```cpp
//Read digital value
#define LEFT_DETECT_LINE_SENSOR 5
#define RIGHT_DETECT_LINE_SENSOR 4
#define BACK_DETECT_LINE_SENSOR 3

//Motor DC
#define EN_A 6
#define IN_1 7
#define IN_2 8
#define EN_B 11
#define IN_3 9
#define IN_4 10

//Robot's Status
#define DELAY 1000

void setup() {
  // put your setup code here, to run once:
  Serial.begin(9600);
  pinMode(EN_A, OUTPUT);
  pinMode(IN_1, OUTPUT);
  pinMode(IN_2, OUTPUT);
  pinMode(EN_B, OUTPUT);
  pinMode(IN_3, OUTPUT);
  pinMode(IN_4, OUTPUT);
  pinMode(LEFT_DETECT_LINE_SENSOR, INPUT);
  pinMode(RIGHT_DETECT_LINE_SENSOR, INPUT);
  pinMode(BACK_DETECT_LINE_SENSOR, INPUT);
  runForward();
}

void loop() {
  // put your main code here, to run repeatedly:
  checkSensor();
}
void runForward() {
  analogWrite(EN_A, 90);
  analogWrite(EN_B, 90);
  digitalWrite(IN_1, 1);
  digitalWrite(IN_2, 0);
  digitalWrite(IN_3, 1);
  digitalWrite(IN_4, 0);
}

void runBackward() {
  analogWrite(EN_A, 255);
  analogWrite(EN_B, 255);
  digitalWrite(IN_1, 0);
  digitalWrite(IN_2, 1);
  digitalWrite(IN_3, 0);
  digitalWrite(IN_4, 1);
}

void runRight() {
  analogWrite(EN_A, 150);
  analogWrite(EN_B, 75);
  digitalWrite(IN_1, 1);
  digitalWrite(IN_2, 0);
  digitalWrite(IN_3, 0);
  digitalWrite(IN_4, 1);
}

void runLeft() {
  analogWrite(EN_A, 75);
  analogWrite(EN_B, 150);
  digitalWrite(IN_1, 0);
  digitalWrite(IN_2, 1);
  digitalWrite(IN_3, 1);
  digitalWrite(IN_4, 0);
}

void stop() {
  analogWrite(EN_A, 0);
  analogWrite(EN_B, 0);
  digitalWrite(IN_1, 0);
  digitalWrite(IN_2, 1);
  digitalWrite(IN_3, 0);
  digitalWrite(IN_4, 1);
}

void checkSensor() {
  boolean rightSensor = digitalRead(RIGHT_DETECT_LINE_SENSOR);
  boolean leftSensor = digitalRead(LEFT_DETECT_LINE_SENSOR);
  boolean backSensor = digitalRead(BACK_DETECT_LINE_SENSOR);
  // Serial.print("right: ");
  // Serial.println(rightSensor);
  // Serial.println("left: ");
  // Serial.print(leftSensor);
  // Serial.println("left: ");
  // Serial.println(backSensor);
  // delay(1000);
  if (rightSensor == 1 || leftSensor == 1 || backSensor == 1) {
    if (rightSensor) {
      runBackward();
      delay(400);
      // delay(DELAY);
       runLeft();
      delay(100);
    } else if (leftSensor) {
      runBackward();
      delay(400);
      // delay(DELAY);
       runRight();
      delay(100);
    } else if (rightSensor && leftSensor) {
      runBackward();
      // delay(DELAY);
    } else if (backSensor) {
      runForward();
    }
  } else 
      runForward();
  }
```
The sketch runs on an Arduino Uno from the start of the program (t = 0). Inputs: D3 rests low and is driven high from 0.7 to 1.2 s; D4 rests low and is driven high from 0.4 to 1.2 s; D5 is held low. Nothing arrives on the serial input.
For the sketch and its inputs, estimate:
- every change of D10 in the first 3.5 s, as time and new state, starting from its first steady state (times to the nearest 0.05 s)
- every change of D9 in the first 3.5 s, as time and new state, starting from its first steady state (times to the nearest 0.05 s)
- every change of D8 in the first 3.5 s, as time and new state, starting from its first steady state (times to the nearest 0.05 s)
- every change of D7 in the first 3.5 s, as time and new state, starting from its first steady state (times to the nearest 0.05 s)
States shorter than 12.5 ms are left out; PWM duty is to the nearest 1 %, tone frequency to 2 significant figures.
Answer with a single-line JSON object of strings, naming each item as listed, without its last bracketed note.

{"every change of D10 in the first 3.5 s, as time and new state, starting from its first steady state": "0 s low; 0.4 s high; 0.8 s low; 0.9 s high; 1.3 s low", "every change of D9 in the first 3.5 s, as time and new state, starting from its first steady state": "0 s high; 0.4 s low; 0.8 s high; 0.9 s low; 1.3 s high", "every change of D8 in the first 3.5 s, as time and new state, starting from its first steady state": "0 s low; 0.4 s high; 1.4 s low", "every change of D7 in the first 3.5 s, as time and new state, starting from its first steady state": "0 s high; 0.4 s low; 1.4 s high"}
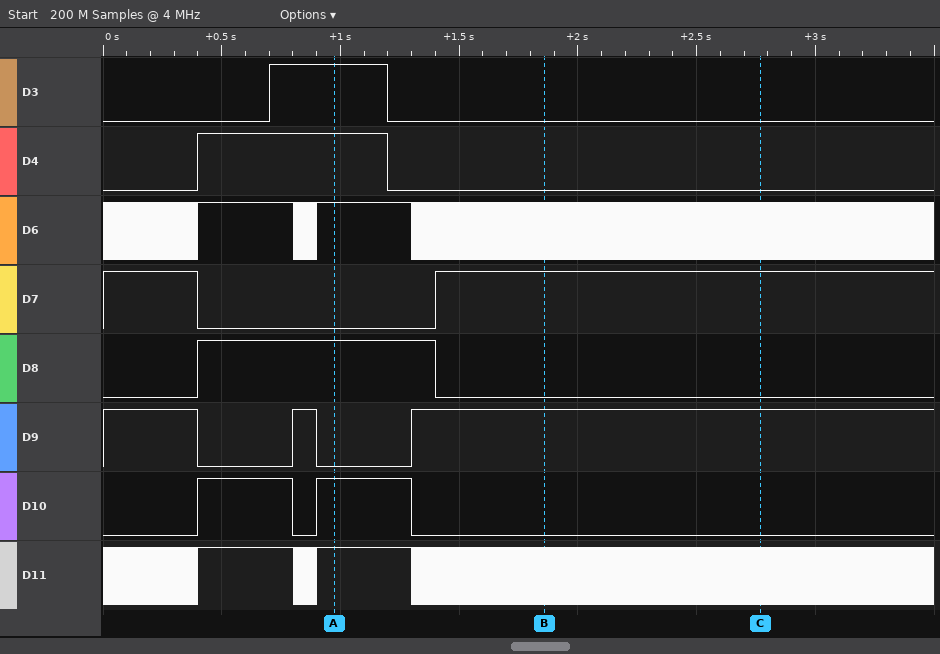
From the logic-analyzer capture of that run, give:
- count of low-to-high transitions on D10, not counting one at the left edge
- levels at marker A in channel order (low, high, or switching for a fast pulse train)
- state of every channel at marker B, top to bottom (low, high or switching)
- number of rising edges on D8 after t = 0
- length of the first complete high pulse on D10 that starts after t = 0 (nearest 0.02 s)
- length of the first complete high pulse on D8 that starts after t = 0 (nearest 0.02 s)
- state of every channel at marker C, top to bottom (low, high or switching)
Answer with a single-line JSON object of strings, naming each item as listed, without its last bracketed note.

{"count of low-to-high transitions on D10, not counting one at the left edge": "2", "levels at marker A in channel order": "D3 high, D4 high, D6 high, D7 low, D8 high, D9 low, D10 high, D11 high", "state of every channel at marker B, top to bottom": "D3 low, D4 low, D6 switching, D7 high, D8 low, D9 high, D10 low, D11 switching", "number of rising edges on D8 after t = 0": "1", "length of the first complete high pulse on D10 that starts after t = 0": "0.40 s", "length of the first complete high pulse on D8 that starts after t = 0": "1.00 s", "state of every channel at marker C, top to bottom": "D3 low, D4 low, D6 switching, D7 high, D8 low, D9 high, D10 low, D11 switching"}
